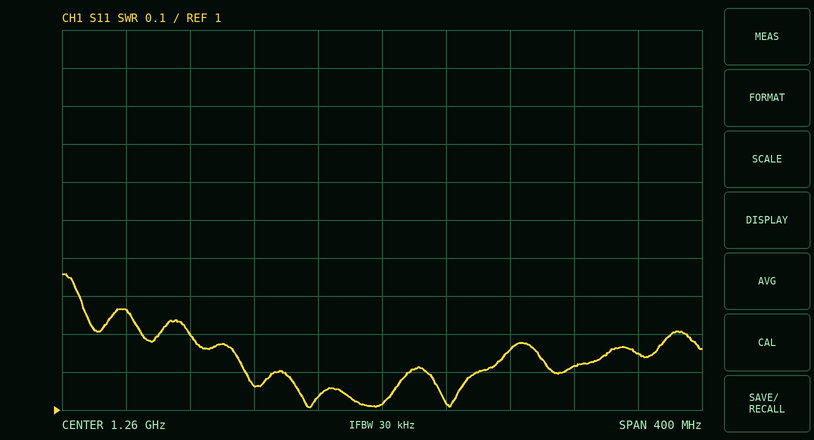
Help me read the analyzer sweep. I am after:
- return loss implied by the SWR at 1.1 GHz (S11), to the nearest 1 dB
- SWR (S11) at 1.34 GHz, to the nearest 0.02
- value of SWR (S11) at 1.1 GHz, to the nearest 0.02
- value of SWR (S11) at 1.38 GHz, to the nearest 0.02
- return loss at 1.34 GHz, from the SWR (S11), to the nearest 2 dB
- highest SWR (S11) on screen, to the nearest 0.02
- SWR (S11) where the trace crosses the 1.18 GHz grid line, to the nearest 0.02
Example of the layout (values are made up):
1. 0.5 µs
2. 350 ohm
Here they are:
1. 19 dB
2. 1.16
3. 1.26
4. 1.12
5. 22 dB
6. 1.36
7. 1.06
